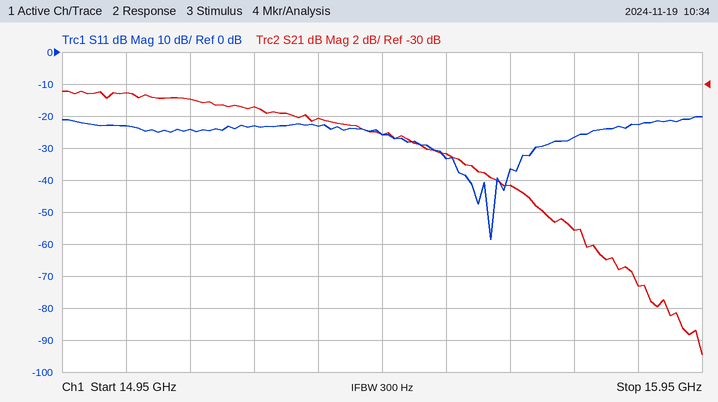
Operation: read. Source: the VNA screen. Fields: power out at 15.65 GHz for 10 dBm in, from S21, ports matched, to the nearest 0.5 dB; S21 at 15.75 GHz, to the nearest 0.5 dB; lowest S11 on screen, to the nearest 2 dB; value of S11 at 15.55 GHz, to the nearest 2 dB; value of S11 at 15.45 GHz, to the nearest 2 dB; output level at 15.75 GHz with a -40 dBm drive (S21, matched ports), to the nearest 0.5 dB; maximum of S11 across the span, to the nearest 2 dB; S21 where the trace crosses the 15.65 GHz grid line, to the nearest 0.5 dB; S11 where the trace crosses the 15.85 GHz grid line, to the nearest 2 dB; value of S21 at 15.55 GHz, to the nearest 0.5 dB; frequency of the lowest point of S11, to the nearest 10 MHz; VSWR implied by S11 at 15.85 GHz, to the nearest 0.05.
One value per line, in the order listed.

-26.5 dBm
-39.0 dB
-58 dB
-34 dB
-26 dB
-79.0 dBm
-20 dB
-36.5 dB
-22 dB
-34.5 dB
15.62 GHz
1.15
